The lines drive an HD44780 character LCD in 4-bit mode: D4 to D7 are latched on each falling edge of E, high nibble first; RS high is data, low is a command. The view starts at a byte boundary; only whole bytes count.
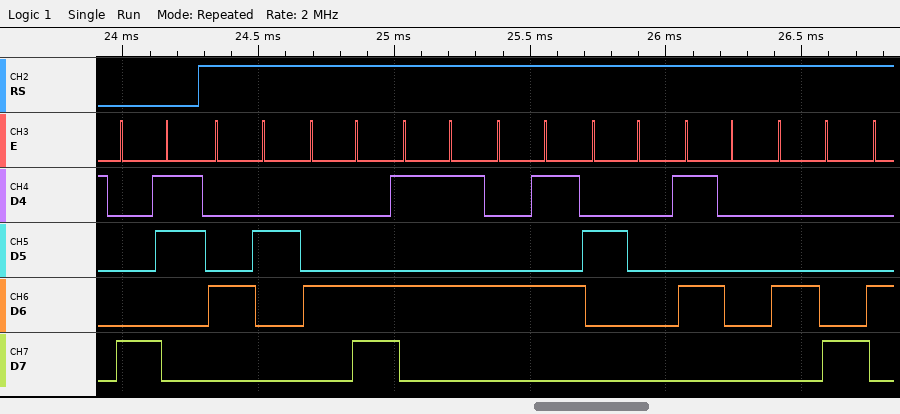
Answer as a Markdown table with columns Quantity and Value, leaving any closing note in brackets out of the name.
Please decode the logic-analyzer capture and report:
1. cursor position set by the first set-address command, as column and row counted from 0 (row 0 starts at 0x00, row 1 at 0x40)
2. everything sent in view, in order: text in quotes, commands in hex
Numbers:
| Quantity | Value |
|---|---|
| cursor position set by the first set-address command, as column and row counted from 0 | column 3, row 0 |
| everything sent in view, in order: text in quotes, commands in hex | 0x83 "BLUE PH" |
